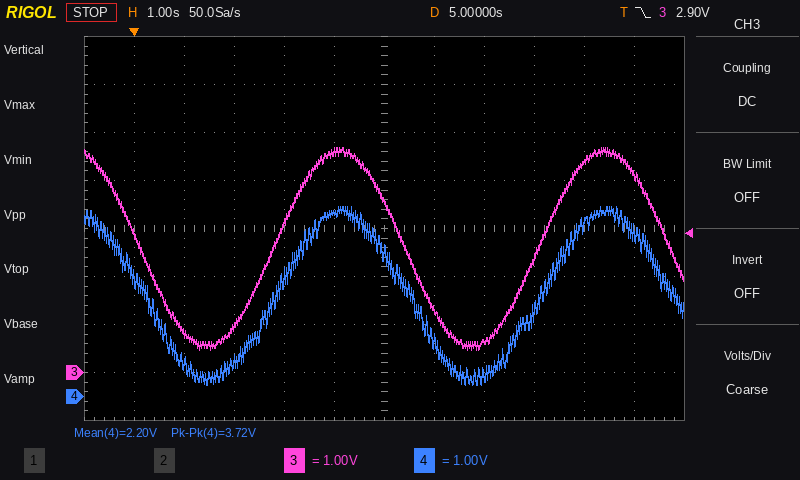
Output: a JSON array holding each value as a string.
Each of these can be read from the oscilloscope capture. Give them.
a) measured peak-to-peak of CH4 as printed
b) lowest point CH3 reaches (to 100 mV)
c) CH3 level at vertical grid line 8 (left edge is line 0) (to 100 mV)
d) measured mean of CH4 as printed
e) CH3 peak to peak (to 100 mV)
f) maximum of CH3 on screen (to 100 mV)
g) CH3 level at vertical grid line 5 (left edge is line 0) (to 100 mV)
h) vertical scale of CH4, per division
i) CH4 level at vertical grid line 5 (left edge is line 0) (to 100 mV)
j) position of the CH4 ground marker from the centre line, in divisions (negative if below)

["3.72 V", "500 mV", "700 mV", "2.20 V", "4.2 V", "4.7 V", "4.6 V", "1 V", "3.8 V", "-3.5 div"]
